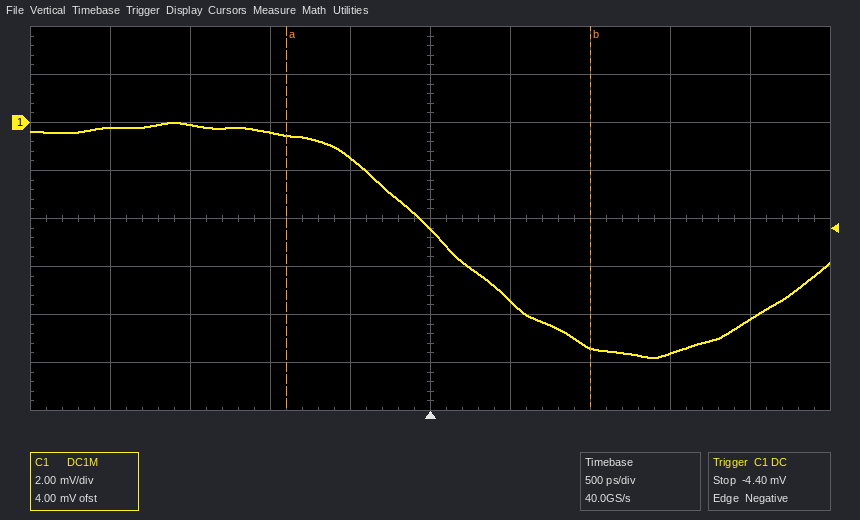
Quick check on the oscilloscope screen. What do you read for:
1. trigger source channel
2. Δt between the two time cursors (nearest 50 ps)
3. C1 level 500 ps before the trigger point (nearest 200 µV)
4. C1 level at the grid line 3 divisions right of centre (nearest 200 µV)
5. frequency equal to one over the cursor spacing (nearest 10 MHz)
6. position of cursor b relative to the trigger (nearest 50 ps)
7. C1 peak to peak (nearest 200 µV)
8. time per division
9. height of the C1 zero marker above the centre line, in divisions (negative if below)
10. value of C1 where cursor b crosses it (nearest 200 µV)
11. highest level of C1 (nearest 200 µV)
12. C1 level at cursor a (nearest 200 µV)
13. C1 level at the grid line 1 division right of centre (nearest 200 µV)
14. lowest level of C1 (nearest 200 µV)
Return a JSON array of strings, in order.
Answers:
["C1", "1.90 ns", "-1.4 mV", "-9.6 mV", "530 MHz", "+1.00 ns", "9.8 mV", "500 ps", "+2.0 div", "-9.4 mV", "0.0 mV", "-600 µV", "-7.4 mV", "-9.8 mV"]
